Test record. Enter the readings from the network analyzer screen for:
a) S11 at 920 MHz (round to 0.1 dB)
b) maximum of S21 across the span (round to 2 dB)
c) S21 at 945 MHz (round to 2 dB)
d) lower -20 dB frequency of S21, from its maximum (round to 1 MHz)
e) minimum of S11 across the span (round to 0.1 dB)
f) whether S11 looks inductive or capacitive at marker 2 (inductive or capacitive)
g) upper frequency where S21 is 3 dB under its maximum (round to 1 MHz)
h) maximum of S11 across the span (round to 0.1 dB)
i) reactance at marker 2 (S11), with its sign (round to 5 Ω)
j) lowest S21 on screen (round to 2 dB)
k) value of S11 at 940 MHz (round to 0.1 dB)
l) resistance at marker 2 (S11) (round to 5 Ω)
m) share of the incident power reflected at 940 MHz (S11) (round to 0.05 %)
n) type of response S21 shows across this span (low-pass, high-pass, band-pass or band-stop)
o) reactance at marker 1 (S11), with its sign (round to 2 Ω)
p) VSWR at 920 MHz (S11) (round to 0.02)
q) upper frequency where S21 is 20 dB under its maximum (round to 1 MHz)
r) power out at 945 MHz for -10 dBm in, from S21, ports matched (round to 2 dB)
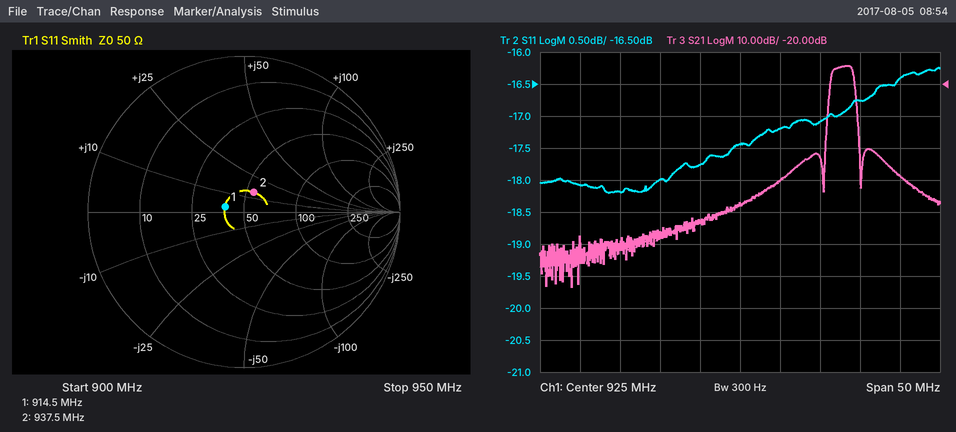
-17.8 dB
-14 dB
-48 dB
936 MHz
-18.2 dB
inductive
939 MHz
-16.2 dB
+15 Ω
-84 dB
-16.8 dB
55 Ω
2.10 %
band-pass
+2 Ω
1.30
940 MHz
-58 dBm
